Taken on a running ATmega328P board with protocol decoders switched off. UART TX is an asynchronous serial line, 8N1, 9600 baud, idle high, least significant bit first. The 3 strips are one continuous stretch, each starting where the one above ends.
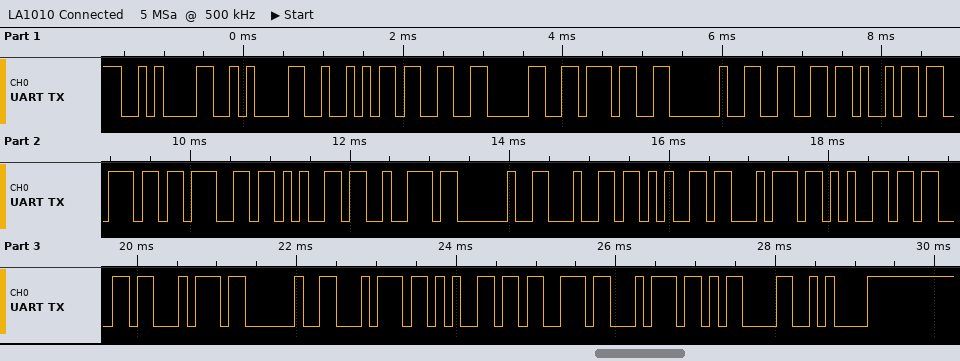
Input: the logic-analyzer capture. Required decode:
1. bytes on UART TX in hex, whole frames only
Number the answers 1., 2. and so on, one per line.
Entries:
1. 0x0A 0x0A 0x52 0x33 0x30 0x37 0x20 0x66 0x69 0x6E 0x67 0x65 0x72 0x20 0x64 0x65 0x74 0x65 0x63 0x74 0x20 0x74 0x65 0x73 0x74 0x0D 0x0A
